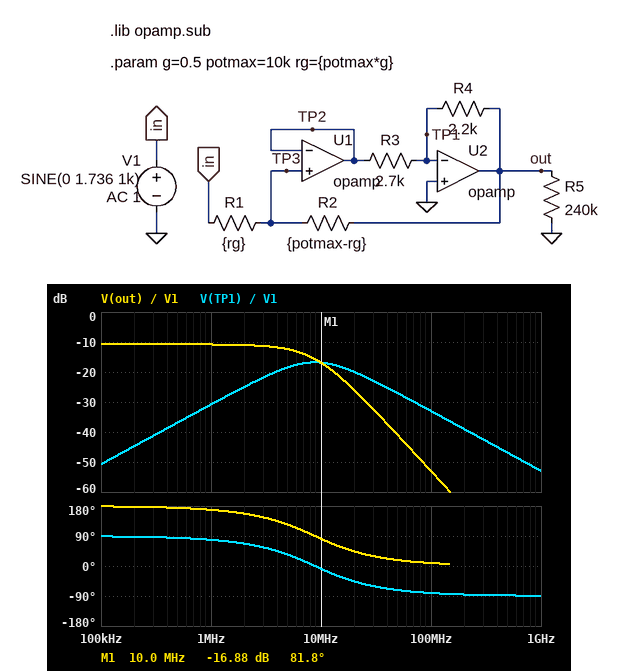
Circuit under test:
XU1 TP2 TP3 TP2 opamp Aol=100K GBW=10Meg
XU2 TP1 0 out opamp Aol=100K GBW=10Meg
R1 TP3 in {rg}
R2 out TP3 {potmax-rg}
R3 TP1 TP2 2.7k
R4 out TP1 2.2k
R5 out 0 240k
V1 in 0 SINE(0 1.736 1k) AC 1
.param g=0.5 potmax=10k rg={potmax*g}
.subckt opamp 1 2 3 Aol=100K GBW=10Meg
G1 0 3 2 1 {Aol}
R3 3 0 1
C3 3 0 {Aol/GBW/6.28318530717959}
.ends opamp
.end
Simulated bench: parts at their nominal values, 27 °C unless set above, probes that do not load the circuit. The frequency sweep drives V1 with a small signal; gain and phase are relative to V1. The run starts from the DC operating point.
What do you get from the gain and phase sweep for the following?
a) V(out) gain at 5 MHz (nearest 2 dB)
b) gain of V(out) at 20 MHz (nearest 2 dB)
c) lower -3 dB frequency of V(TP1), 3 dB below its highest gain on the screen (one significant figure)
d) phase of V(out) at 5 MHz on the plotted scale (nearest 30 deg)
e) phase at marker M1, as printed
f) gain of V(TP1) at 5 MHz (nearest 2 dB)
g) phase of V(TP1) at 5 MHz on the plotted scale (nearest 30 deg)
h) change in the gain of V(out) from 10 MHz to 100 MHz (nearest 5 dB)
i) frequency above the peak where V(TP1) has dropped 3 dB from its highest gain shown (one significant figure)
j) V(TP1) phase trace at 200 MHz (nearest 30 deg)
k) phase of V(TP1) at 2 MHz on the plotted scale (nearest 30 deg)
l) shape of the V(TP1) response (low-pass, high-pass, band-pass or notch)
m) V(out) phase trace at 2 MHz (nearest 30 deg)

-12 dB
-26 dB
4 MHz
120 deg
81.8 deg
-18 dB
30 deg
-35 dB
20 MHz
-90 deg
60 deg
band-pass
150 deg
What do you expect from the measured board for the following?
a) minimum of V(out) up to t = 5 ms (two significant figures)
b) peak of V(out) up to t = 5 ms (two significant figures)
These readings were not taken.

-500 mV
500 mV
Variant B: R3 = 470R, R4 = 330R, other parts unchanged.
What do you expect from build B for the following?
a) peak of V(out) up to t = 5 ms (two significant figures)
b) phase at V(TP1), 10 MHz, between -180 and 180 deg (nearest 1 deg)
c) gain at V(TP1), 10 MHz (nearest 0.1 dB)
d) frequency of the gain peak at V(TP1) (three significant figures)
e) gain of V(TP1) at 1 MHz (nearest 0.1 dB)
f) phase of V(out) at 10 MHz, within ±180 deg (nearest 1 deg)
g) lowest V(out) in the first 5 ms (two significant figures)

450 mV
-7 deg
-17.8 dB
8.91 MHz
-31.8 dB
83 deg
-450 mV
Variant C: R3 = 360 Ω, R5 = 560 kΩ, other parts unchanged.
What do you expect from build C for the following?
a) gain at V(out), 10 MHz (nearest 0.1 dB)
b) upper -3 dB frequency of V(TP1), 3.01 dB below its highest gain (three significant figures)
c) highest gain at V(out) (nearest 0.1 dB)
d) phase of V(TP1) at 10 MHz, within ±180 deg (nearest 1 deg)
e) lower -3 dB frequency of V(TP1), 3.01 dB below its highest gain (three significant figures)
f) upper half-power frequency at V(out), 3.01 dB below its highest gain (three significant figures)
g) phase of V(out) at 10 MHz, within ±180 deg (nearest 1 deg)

-9.1 dB
15.2 MHz
-2.5 dB
-21 deg
3.76 MHz
7.04 MHz
69 deg
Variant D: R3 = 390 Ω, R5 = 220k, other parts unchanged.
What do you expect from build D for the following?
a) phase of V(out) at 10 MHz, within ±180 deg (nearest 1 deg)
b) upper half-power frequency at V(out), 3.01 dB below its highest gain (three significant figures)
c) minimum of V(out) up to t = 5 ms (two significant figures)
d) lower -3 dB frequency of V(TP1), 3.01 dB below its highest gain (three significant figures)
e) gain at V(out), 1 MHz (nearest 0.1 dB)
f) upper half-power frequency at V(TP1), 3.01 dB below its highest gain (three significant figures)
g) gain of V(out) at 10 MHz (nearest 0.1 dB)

70 deg
7.04 MHz
-1.3 V
3.77 MHz
-2.7 dB
15.3 MHz
-9.2 dB
